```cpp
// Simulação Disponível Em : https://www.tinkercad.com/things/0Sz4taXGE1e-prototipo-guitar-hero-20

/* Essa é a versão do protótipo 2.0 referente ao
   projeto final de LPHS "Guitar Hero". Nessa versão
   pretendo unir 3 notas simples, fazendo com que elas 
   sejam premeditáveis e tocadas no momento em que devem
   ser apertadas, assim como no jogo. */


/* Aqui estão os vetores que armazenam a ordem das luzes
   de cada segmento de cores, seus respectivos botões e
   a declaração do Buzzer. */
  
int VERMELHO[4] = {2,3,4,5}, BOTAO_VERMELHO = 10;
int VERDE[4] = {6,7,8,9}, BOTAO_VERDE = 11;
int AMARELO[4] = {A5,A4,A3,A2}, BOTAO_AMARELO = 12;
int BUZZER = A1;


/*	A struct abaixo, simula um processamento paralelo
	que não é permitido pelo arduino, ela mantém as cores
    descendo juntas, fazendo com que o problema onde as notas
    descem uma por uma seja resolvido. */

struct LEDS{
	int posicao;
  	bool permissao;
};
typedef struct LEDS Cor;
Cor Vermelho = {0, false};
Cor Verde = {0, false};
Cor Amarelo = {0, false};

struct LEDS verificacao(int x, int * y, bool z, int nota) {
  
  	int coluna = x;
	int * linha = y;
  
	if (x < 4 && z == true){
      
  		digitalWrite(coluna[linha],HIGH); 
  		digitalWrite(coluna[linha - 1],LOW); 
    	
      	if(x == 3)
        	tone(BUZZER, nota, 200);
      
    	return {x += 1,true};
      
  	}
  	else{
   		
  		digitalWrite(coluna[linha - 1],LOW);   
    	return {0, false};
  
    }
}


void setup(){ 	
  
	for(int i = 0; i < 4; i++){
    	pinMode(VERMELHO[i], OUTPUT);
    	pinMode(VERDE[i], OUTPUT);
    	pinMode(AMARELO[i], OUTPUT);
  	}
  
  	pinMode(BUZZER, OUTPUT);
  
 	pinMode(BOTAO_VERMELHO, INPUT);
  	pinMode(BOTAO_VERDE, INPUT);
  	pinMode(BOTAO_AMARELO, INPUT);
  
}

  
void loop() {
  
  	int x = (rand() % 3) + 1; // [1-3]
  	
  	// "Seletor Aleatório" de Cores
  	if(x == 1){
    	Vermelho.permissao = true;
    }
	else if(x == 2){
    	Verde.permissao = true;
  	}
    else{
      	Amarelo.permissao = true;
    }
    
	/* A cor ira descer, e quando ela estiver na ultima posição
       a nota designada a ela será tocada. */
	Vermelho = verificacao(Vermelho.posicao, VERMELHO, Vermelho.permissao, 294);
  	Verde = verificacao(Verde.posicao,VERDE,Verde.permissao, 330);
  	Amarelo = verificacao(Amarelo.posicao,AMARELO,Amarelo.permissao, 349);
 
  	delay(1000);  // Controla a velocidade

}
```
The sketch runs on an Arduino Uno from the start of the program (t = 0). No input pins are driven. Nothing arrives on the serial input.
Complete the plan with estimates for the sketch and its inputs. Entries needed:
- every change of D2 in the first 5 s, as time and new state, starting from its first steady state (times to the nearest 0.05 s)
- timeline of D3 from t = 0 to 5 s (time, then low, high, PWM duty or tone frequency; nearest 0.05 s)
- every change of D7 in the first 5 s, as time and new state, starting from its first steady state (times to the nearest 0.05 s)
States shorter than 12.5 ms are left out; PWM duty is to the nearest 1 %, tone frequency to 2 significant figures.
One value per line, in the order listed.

0 s low; 2 s high; 3 s low
0 s low; 3 s high; 4 s low
0 s low; 1 s high; 2 s low
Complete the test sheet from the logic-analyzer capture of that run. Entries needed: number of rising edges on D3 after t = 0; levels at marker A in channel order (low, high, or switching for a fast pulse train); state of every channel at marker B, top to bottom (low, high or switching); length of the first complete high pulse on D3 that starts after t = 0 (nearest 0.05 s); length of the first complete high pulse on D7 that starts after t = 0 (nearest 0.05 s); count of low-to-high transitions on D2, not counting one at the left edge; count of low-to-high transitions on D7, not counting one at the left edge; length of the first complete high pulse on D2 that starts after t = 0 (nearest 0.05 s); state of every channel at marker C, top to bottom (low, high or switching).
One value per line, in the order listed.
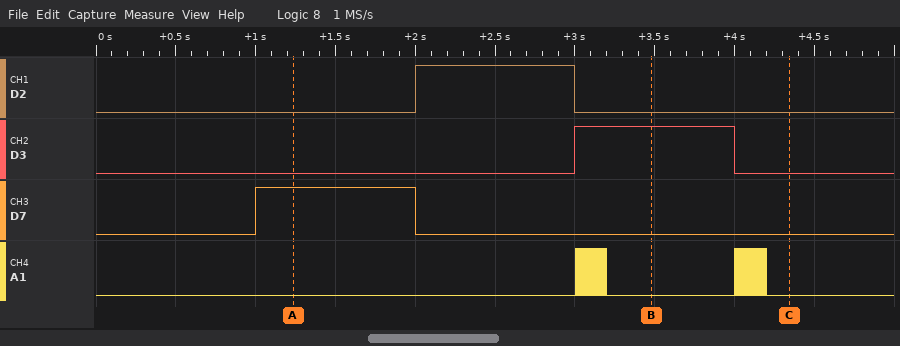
1
D2 low, D3 low, D7 high, A1 low
D2 low, D3 high, D7 low, A1 low
1.00 s
1.00 s
1
1
1.00 s
D2 low, D3 low, D7 low, A1 low
